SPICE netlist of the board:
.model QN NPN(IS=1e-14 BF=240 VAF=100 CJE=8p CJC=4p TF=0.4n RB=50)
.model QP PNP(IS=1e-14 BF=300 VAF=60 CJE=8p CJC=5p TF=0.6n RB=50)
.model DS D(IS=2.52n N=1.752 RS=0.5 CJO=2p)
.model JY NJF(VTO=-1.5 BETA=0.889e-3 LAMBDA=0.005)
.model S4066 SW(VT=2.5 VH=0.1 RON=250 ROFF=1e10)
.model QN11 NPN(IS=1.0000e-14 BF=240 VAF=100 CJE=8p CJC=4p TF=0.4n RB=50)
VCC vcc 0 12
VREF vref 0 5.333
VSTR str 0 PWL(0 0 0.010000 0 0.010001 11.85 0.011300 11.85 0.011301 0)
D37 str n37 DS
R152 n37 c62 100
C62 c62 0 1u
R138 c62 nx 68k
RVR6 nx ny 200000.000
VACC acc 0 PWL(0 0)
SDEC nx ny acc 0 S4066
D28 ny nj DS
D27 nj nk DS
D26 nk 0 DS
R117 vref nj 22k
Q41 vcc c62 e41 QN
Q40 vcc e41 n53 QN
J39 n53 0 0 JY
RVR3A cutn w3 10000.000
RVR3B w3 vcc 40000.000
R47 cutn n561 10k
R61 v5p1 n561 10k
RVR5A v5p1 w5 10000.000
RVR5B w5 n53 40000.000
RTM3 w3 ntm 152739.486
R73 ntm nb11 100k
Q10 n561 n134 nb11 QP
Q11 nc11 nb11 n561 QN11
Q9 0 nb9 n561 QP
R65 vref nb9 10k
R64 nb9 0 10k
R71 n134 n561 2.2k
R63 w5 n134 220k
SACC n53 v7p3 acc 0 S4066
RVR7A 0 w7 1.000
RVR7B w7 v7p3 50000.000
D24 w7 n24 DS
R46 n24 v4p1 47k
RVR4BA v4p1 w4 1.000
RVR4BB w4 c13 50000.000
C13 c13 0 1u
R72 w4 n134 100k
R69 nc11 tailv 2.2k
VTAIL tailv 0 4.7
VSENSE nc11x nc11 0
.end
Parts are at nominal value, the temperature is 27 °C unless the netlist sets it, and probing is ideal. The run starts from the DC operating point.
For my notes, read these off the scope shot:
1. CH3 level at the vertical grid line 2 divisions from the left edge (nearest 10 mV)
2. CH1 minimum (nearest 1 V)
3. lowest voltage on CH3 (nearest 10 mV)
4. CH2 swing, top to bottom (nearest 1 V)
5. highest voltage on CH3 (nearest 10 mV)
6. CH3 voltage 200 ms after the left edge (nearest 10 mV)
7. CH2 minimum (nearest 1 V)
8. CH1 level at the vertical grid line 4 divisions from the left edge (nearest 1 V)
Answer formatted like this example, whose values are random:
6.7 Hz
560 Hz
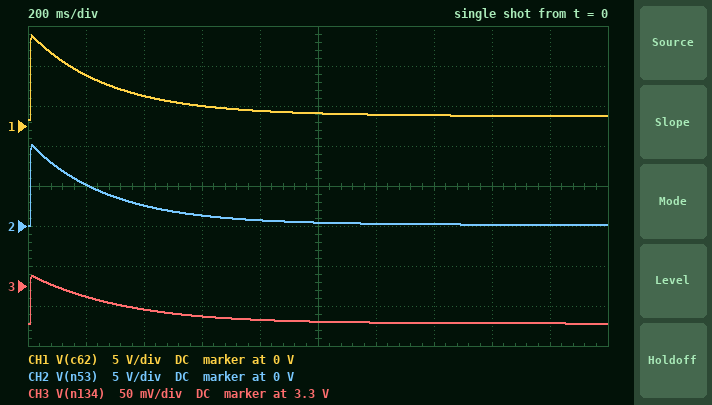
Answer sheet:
3.27 V
1 V
3.25 V
10 V
3.31 V
3.29 V
0 V
2 V
